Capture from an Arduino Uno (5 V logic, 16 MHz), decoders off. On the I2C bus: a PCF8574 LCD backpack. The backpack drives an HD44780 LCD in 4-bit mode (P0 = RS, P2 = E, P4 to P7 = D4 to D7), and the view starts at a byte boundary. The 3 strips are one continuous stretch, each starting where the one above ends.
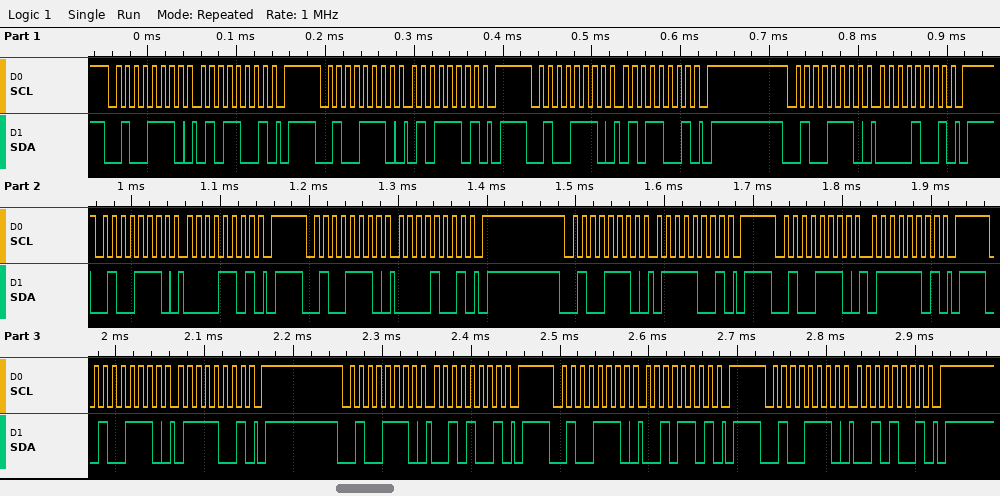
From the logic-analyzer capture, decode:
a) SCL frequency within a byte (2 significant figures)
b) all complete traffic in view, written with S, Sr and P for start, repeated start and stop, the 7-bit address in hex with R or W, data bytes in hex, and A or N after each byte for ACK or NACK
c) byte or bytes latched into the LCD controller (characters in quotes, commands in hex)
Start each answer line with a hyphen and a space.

- 100 kHz
- S 27W A 59 A P S 27W A 5D A P S 27W A 59 A P S 27W A 09 A P S 27W A 0D A P S 27W A 09 A P S 27W A 79 A P S 27W A 7D A P S 27W A 79 A P S 27W A 29 A P S 27W A 2D A P S 27W A 29 A P
- 'P' 'r'
